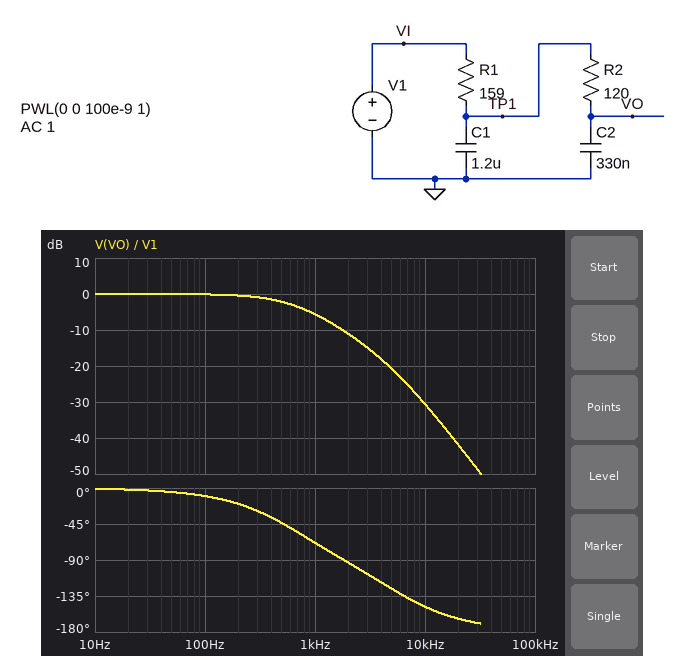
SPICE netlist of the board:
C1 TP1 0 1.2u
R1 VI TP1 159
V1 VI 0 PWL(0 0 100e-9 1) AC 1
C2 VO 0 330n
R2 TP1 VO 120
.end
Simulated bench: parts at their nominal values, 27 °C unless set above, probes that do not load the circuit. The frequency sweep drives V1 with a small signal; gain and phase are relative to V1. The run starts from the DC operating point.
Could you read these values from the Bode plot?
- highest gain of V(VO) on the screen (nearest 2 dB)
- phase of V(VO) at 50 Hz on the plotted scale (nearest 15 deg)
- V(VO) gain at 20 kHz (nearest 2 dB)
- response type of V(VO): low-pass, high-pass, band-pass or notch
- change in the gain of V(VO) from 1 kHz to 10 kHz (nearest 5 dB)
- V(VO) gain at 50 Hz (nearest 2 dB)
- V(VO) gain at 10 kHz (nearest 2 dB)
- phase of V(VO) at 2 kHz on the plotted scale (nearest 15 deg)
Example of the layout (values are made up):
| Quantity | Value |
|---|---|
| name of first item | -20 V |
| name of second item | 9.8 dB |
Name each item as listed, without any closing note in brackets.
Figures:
| Quantity | Value |
|---|---|
| highest gain of V(VO) on the screen | 0 dB |
| phase of V(VO) at 50 Hz on the plotted scale | 0 deg |
| V(VO) gain at 20 kHz | -42 dB |
| response type of V(VO): low-pass, high-pass, band-pass or notch | low-pass |
| change in the gain of V(VO) from 1 kHz to 10 kHz | -25 dB |
| V(VO) gain at 50 Hz | 0 dB |
| V(VO) gain at 10 kHz | -30 dB |
| phase of V(VO) at 2 kHz on the plotted scale | -90 deg |
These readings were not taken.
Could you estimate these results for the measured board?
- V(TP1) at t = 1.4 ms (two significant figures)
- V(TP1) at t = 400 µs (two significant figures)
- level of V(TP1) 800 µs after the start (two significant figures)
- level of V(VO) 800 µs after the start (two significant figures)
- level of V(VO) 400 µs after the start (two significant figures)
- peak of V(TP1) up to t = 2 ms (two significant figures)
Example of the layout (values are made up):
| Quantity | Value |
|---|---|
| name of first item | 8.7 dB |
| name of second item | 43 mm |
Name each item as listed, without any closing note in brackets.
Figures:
| Quantity | Value |
|---|---|
| V(TP1) at t = 1.4 ms | 1.0 V |
| V(TP1) at t = 400 µs | 800 mV |
| level of V(TP1) 800 µs after the start | 960 mV |
| level of V(VO) 800 µs after the start | 950 mV |
| level of V(VO) 400 µs after the start | 770 mV |
| peak of V(TP1) up to t = 2 ms | 1.0 V |
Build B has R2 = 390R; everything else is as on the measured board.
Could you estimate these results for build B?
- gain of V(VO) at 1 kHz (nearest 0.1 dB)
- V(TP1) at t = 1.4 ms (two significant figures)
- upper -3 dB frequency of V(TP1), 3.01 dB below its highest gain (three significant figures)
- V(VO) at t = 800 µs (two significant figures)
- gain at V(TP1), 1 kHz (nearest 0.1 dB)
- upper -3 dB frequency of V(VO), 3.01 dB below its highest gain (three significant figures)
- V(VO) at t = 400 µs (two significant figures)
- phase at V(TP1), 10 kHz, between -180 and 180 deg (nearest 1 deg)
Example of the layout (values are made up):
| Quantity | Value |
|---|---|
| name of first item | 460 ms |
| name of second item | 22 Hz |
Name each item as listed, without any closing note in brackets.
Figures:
| Quantity | Value |
|---|---|
| gain of V(VO) at 1 kHz | -7.4 dB |
| V(TP1) at t = 1.4 ms | 990 mV |
| upper -3 dB frequency of V(TP1), 3.01 dB below its highest gain | 623 Hz |
| V(VO) at t = 800 µs | 910 mV |
| gain at V(TP1), 1 kHz | -5.2 dB |
| upper -3 dB frequency of V(VO), 3.01 dB below its highest gain | 515 Hz |
| V(VO) at t = 400 µs | 650 mV |
| phase at V(TP1), 10 kHz, between -180 and 180 deg | -83 deg |
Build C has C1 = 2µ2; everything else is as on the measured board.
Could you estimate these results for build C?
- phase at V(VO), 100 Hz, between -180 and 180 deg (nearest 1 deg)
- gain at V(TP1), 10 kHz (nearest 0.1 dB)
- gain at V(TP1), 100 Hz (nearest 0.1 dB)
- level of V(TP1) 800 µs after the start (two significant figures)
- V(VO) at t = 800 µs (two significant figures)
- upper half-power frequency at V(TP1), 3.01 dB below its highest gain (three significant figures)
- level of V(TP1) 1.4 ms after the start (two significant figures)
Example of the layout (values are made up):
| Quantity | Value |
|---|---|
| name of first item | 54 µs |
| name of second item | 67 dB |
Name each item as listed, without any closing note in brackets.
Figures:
| Quantity | Value |
|---|---|
| phase at V(VO), 100 Hz, between -180 and 180 deg | -16 deg |
| gain at V(TP1), 10 kHz | -27.1 dB |
| gain at V(TP1), 100 Hz | -0.3 dB |
| level of V(TP1) 800 µs after the start | 860 mV |
| V(VO) at t = 800 µs | 850 mV |
| upper half-power frequency at V(TP1), 3.01 dB below its highest gain | 391 Hz |
| level of V(TP1) 1.4 ms after the start | 970 mV |
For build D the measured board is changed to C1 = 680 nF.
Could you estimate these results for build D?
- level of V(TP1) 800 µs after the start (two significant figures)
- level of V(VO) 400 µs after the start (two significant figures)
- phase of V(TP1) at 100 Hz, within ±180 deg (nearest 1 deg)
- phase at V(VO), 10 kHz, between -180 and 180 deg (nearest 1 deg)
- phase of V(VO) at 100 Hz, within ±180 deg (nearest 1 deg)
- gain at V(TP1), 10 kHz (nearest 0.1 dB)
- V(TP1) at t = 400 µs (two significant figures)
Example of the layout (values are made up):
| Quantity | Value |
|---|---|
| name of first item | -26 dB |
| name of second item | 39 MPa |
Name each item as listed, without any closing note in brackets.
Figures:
| Quantity | Value |
|---|---|
| level of V(TP1) 800 µs after the start | 990 mV |
| level of V(VO) 400 µs after the start | 880 mV |
| phase of V(TP1) at 100 Hz, within ±180 deg | -6 deg |
| phase at V(VO), 10 kHz, between -180 and 180 deg | -142 deg |
| phase of V(VO) at 100 Hz, within ±180 deg | -7 deg |
| gain at V(TP1), 10 kHz | -17.6 dB |
| V(TP1) at t = 400 µs | 910 mV |
